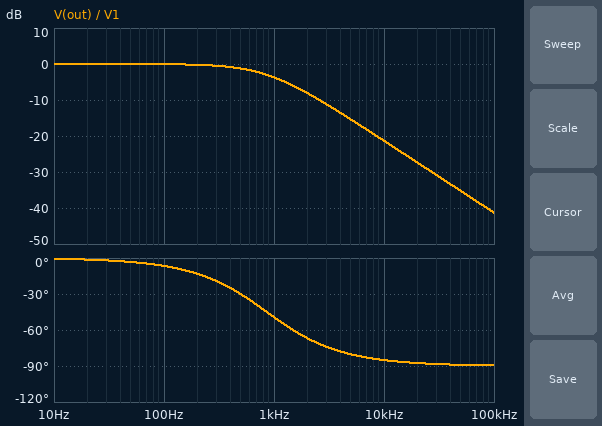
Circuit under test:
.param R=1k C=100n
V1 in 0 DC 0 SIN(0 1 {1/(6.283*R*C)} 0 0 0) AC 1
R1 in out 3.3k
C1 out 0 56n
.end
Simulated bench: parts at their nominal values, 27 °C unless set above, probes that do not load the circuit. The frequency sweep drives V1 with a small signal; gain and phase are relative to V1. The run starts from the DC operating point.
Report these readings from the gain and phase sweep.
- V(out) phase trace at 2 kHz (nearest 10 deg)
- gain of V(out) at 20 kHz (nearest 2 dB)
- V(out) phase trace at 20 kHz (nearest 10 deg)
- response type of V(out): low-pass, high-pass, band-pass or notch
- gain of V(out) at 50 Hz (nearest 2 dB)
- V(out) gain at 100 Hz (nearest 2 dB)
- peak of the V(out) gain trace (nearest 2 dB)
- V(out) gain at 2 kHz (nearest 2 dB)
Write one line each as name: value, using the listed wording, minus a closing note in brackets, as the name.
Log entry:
V(out) phase trace at 2 kHz: -70 deg
gain of V(out) at 20 kHz: -28 dB
V(out) phase trace at 20 kHz: -90 deg
response type of V(out): low-pass, high-pass, band-pass or notch: low-pass
gain of V(out) at 50 Hz: 0 dB
V(out) gain at 100 Hz: 0 dB
peak of the V(out) gain trace: 0 dB
V(out) gain at 2 kHz: -8 dB
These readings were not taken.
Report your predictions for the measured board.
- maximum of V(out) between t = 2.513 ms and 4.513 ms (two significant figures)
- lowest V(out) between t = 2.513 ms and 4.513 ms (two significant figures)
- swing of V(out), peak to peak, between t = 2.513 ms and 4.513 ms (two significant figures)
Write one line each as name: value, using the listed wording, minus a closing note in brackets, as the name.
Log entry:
maximum of V(out) between t = 2.513 ms and 4.513 ms: 480 mV
lowest V(out) between t = 2.513 ms and 4.513 ms: -480 mV
swing of V(out), peak to peak, between t = 2.513 ms and 4.513 ms: 950 mV
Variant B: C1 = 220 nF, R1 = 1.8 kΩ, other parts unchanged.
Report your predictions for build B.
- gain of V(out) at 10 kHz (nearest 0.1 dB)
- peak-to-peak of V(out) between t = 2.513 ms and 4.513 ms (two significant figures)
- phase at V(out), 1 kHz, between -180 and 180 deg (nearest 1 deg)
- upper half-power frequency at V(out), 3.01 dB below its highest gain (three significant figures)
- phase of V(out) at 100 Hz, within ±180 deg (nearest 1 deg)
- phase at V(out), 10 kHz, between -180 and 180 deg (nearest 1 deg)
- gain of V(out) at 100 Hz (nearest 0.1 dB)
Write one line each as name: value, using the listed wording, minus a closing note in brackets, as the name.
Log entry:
gain of V(out) at 10 kHz: -27.9 dB
peak-to-peak of V(out) between t = 2.513 ms and 4.513 ms: 490 mV
phase at V(out), 1 kHz, between -180 and 180 deg: -68 deg
upper half-power frequency at V(out), 3.01 dB below its highest gain: 402 Hz
phase of V(out) at 100 Hz, within ±180 deg: -14 deg
phase at V(out), 10 kHz, between -180 and 180 deg: -88 deg
gain of V(out) at 100 Hz: -0.3 dB
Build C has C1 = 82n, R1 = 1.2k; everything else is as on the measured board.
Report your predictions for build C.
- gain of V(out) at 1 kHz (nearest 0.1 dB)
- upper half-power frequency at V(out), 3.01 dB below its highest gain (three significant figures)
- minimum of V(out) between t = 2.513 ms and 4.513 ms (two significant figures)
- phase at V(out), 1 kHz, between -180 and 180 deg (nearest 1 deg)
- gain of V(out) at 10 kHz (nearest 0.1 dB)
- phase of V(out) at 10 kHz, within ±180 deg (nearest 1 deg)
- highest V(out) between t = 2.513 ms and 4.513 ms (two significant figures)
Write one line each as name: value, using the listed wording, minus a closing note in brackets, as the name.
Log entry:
gain of V(out) at 1 kHz: -1.4 dB
upper half-power frequency at V(out), 3.01 dB below its highest gain: 1.62 kHz
minimum of V(out) between t = 2.513 ms and 4.513 ms: -710 mV
phase at V(out), 1 kHz, between -180 and 180 deg: -32 deg
gain of V(out) at 10 kHz: -15.9 dB
phase of V(out) at 10 kHz, within ±180 deg: -81 deg
highest V(out) between t = 2.513 ms and 4.513 ms: 710 mV
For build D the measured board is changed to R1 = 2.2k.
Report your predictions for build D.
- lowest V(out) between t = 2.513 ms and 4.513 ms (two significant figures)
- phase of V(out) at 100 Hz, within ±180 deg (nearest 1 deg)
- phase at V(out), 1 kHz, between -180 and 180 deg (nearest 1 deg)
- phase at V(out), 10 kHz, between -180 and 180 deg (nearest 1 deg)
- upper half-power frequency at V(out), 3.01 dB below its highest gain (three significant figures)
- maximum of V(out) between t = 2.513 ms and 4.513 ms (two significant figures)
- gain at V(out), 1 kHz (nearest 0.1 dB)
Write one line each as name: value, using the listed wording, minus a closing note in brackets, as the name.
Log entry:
lowest V(out) between t = 2.513 ms and 4.513 ms: -630 mV
phase of V(out) at 100 Hz, within ±180 deg: -4 deg
phase at V(out), 1 kHz, between -180 and 180 deg: -38 deg
phase at V(out), 10 kHz, between -180 and 180 deg: -83 deg
upper half-power frequency at V(out), 3.01 dB below its highest gain: 1.29 kHz
maximum of V(out) between t = 2.513 ms and 4.513 ms: 630 mV
gain at V(out), 1 kHz: -2.0 dB
